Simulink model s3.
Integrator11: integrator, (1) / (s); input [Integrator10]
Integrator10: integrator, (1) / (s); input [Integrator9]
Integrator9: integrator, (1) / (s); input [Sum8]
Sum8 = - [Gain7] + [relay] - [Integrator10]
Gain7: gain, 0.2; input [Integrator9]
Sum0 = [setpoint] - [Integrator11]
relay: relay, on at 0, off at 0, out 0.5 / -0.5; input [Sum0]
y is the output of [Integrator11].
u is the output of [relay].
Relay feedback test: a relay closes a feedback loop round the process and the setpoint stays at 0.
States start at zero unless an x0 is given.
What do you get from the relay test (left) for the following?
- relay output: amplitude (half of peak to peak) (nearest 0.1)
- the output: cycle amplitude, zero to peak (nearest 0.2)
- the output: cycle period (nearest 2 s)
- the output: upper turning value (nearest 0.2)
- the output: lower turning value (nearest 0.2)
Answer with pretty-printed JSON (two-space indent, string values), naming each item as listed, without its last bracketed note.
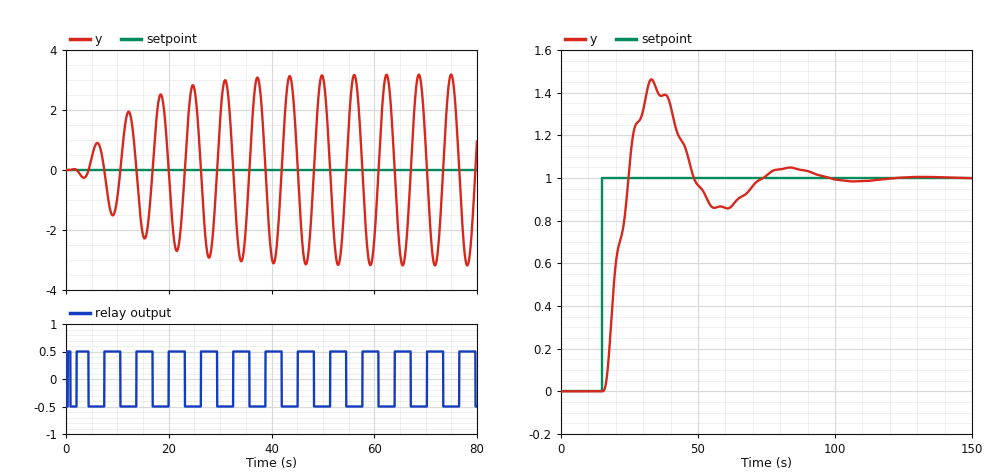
{
  "relay output: amplitude (half of peak to peak)": "0.5",
  "the output: cycle amplitude, zero to peak": "3.2",
  "the output: cycle period": "6 s",
  "the output: upper turning value": "3.2",
  "the output: lower turning value": "-3.2"
}
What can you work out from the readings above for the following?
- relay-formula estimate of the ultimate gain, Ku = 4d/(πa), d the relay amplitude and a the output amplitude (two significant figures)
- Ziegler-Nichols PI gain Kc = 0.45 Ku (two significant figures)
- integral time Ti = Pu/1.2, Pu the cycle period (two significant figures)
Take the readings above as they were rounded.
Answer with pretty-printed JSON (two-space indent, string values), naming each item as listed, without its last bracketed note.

{
  "relay-formula estimate of the ultimate gain, Ku = 4d/(πa), d the relay amplitude and a the output amplitude": "0.20",
  "Ziegler-Nichols PI gain Kc = 0.45 Ku": "0.090",
  "integral time Ti = Pu/1.2, Pu the cycle period": "5.0 s"
}
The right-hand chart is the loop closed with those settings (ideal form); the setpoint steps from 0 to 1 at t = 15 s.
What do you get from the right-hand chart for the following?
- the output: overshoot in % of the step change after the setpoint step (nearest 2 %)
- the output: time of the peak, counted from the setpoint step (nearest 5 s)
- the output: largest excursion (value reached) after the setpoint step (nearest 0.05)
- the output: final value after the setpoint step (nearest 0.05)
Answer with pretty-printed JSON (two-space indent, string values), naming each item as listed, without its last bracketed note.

{
  "the output: overshoot in % of the step change after the setpoint step": "46 %",
  "the output: time of the peak, counted from the setpoint step": "20 s",
  "the output: largest excursion (value reached) after the setpoint step": "1.45",
  "the output: final value after the setpoint step": "1.00"
}
